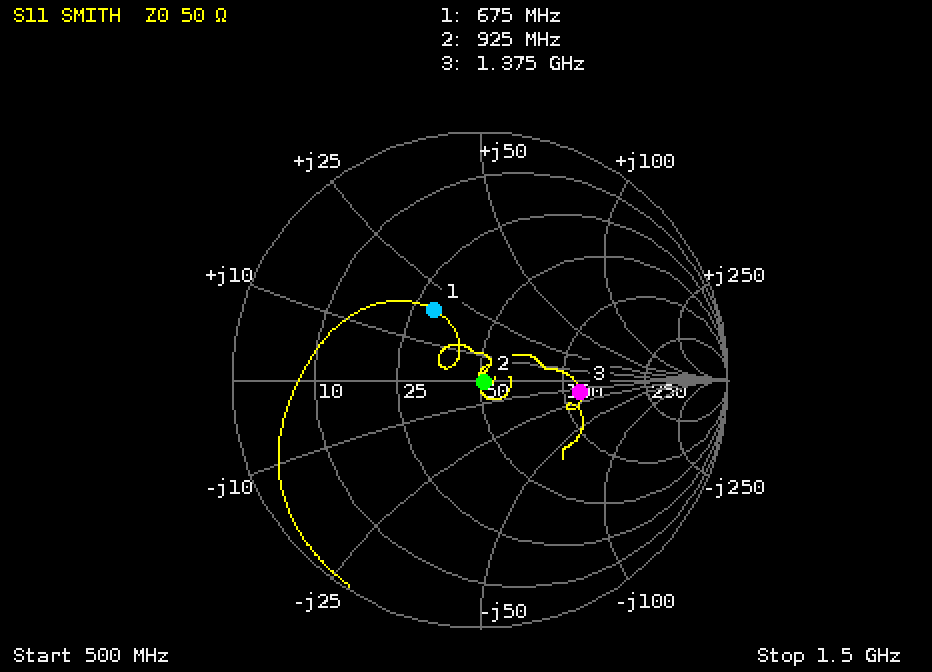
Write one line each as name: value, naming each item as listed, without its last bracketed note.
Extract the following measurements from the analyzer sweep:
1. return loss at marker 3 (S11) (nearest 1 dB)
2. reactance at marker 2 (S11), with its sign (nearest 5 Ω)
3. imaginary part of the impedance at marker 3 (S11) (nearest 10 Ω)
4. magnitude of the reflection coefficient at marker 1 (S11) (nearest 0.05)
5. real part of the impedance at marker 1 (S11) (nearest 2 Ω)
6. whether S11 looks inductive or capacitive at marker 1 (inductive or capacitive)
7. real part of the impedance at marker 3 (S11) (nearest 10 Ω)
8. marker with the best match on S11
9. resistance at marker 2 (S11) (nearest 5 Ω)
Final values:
return loss at marker 3 (S11): 8 dB
reactance at marker 2 (S11), with its sign: 0 Ω
imaginary part of the impedance at marker 3 (S11): -10 Ω
magnitude of the reflection coefficient at marker 1 (S11): 0.35
real part of the impedance at marker 1 (S11): 30 Ω
whether S11 looks inductive or capacitive at marker 1: inductive
real part of the impedance at marker 3 (S11): 120 Ω
marker with the best match on S11: marker 2
resistance at marker 2 (S11): 50 Ω
